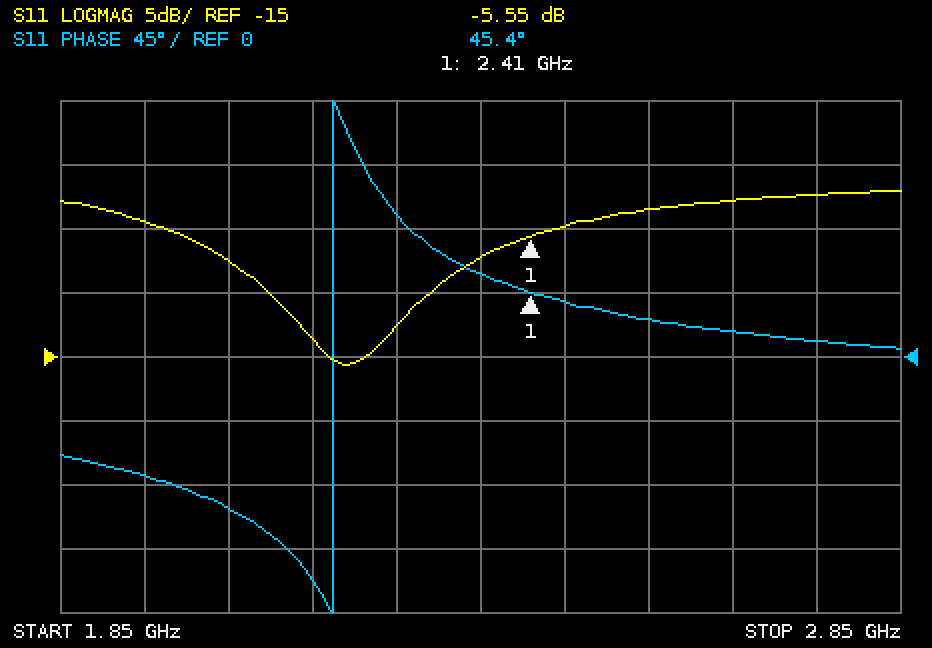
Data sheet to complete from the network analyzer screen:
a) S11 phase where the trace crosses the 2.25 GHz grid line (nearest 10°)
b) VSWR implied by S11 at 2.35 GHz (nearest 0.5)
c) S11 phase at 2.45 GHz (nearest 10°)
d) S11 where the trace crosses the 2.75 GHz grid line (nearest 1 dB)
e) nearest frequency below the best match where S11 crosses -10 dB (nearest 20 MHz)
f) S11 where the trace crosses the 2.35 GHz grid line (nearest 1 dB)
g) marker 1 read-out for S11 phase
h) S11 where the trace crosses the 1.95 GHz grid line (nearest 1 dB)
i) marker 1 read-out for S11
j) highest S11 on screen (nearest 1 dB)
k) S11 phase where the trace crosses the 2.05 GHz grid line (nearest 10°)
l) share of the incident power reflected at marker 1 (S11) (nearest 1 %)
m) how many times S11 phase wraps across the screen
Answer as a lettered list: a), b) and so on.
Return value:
a) 100°
b) 2.5
c) 40°
d) -2 dB
e) 2.10 GHz
f) -7 dB
g) 45.4°
h) -4 dB
i) -5.55 dB
j) -2 dB
k) -110°
l) 28 %
m) 1
